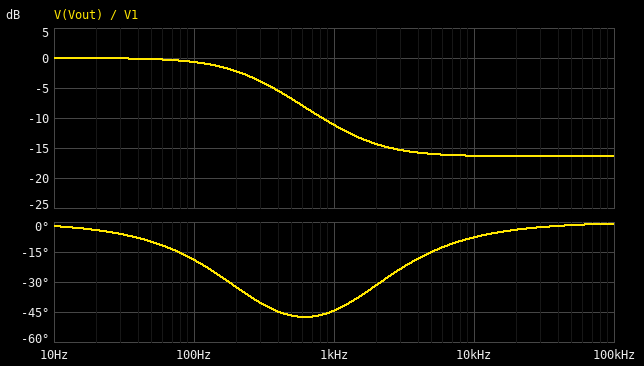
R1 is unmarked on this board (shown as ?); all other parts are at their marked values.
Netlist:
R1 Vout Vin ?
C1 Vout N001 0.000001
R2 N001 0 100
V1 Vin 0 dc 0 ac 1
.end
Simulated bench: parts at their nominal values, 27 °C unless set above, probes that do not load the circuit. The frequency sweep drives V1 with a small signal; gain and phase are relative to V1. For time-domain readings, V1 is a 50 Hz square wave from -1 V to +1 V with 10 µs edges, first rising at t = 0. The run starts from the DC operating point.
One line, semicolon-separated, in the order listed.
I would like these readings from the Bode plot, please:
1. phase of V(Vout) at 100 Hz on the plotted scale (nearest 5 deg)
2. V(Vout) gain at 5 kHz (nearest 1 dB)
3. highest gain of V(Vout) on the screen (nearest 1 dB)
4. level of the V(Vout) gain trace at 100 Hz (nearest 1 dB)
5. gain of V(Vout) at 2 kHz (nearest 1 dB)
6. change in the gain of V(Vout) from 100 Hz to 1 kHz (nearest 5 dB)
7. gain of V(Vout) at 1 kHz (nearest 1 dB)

-20 deg; -16 dB; 0 dB; -1 dB; -14 dB; -10 dB; -11 dB
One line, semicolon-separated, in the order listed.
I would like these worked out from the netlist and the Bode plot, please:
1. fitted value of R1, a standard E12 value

560 Ω
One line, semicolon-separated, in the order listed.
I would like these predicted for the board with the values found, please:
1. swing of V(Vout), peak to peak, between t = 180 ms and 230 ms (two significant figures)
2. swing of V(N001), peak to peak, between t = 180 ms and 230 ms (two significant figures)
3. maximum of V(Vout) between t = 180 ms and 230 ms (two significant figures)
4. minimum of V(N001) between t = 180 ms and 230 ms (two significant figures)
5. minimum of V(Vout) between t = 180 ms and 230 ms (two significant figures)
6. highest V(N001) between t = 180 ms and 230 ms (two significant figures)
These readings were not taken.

2.0 V; 600 mV; 1.0 V; -300 mV; -1.0 V; 300 mV
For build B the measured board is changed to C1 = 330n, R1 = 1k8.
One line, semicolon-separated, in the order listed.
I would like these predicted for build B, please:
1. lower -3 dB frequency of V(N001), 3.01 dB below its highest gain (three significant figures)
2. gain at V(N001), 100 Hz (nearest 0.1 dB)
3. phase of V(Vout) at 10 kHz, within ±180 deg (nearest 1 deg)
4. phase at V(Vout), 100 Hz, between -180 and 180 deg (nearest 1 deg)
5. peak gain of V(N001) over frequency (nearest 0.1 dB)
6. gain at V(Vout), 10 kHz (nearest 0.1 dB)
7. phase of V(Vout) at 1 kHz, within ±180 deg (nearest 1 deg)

254 Hz; -34.3 dB; -24 deg; -20 deg; -25.6 dB; -24.7 dB; -64 deg
